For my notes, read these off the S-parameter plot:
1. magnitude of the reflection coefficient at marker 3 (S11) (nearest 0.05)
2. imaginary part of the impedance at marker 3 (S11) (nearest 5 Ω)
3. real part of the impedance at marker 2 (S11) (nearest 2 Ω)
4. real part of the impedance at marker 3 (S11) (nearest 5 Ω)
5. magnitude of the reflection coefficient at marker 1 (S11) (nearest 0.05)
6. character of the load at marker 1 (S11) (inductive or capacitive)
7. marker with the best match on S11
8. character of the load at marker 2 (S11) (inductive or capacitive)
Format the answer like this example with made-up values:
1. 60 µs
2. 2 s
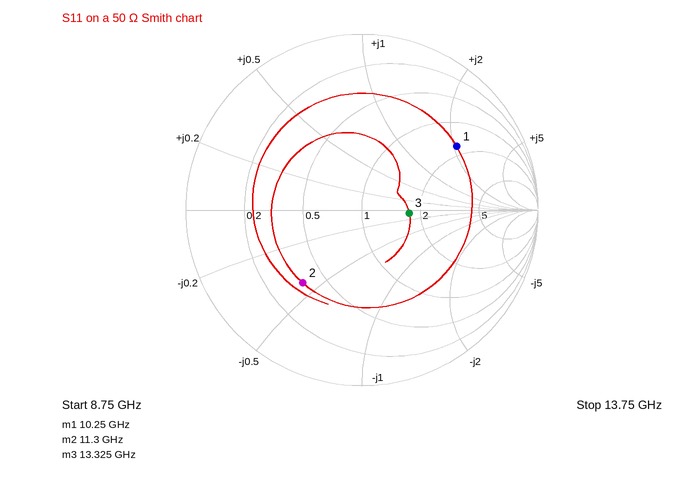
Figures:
1. 0.25
2. -5 Ω
3. 18 Ω
4. 85 Ω
5. 0.65
6. inductive
7. marker 3
8. capacitive
